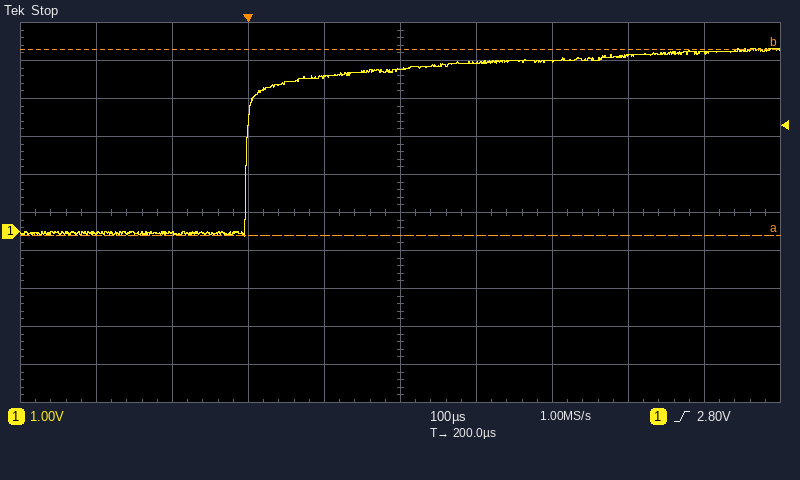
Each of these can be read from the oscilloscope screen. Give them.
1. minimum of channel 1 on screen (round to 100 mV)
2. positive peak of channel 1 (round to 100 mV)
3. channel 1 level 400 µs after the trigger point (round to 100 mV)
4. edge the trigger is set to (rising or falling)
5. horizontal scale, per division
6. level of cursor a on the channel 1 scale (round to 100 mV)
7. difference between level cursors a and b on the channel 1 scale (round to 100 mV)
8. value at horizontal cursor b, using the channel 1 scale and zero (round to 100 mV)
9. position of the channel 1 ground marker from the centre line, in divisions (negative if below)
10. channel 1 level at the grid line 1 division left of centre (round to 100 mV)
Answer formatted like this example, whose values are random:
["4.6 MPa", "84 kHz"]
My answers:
["-100 mV", "4.8 V", "4.5 V", "rising", "100 µs", "-100 mV", "4.9 V", "4.8 V", "-0.5 div", "4.1 V"]
